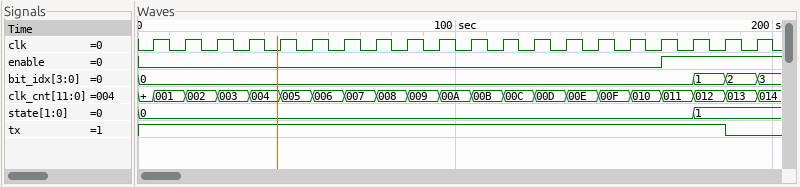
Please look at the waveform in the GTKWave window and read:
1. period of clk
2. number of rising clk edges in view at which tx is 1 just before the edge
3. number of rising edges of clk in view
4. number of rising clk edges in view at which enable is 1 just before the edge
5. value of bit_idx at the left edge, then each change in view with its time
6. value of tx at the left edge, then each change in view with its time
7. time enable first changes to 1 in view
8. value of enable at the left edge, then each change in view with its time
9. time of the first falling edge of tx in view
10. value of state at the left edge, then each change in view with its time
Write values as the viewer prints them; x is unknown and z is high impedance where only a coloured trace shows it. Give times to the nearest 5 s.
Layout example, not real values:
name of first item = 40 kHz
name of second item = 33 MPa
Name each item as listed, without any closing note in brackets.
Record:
period of clk = 10 s
number of rising clk edges in view at which tx is 1 just before the edge = 19
number of rising edges of clk in view = 20
number of rising clk edges in view at which enable is 1 just before the edge = 3
value of bit_idx at the left edge, then each change in view with its time = 0, 1 at 175 s, 2 at 185 s, 3 at 195 s
value of tx at the left edge, then each change in view with its time = 1, 0 at 185 s
time enable first changes to 1 in view = 165 s
value of enable at the left edge, then each change in view with its time = 0, 1 at 165 s
time of the first falling edge of tx in view = 185 s
value of state at the left edge, then each change in view with its time = 0, 1 at 175 s
